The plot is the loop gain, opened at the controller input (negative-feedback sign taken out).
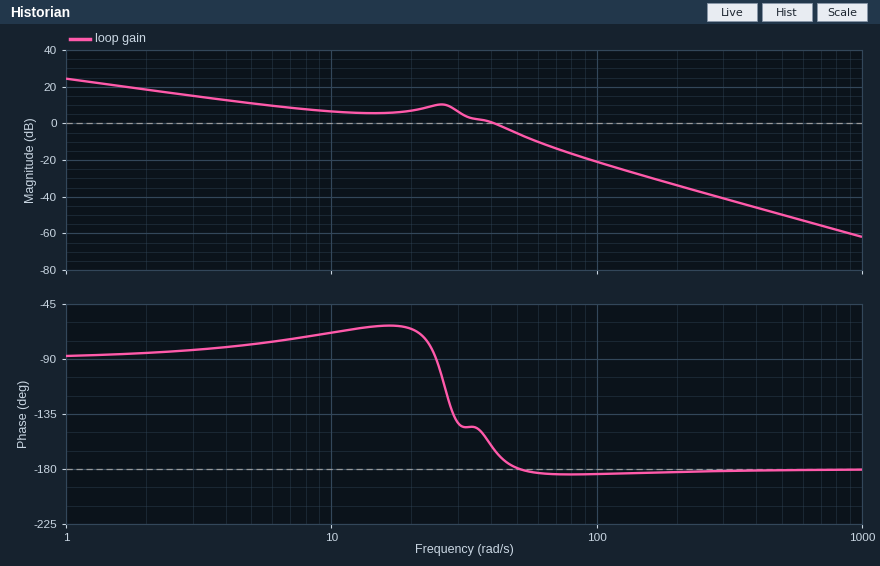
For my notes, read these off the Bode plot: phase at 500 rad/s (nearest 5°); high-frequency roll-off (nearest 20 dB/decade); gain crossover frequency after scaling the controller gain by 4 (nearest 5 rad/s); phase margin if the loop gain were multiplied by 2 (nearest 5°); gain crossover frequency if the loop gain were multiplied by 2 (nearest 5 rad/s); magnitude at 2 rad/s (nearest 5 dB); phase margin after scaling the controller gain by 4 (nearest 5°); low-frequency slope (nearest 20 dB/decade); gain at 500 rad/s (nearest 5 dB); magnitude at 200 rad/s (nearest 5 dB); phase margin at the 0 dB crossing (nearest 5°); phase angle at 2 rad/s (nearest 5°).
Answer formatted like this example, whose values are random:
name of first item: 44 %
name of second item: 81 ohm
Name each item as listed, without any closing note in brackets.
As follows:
phase at 500 rad/s: -180°
high-frequency roll-off: -40 dB/decade
gain crossover frequency after scaling the controller gain by 4: 65 rad/s
phase margin if the loop gain were multiplied by 2: 0°
gain crossover frequency if the loop gain were multiplied by 2: 50 rad/s
magnitude at 2 rad/s: 20 dB
phase margin after scaling the controller gain by 4: -5°
low-frequency slope: -20 dB/decade
gain at 500 rad/s: -50 dB
magnitude at 200 rad/s: -35 dB
phase margin at the 0 dB crossing: 15°
phase angle at 2 rad/s: -85°
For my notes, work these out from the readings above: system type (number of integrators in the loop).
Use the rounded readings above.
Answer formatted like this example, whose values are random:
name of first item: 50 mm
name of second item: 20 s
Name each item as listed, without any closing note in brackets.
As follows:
system type: 1
